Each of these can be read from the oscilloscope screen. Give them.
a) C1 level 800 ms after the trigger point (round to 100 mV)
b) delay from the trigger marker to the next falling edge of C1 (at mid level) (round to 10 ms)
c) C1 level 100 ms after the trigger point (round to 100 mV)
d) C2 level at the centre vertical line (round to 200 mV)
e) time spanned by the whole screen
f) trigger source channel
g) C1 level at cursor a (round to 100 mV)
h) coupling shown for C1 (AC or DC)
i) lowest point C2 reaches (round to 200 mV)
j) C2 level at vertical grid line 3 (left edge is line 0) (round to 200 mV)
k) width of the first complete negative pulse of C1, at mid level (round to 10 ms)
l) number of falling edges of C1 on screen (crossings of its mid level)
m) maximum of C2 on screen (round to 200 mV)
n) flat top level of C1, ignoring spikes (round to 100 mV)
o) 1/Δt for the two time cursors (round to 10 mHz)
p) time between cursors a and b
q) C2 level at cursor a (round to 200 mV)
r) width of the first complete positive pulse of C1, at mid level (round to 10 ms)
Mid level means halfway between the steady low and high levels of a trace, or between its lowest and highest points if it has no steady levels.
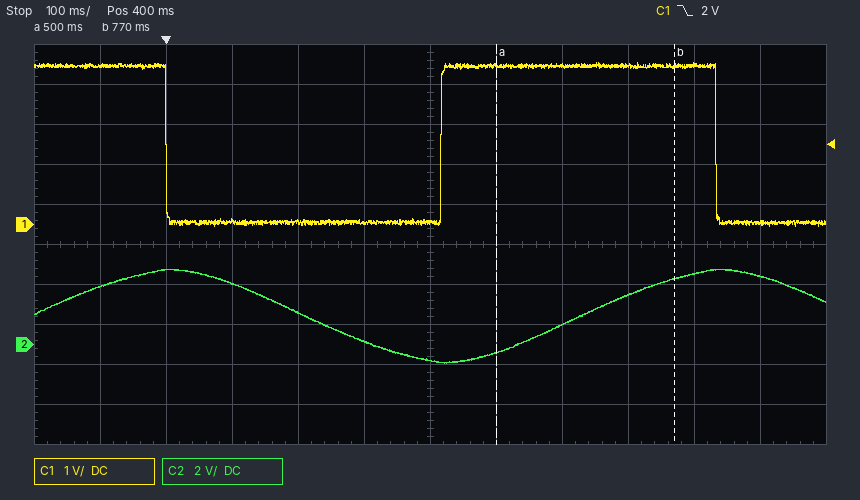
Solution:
4.0 V
830 ms
100 mV
-800 mV
1.2 s
C1
4.0 V
DC
-1.0 V
3.0 V
420 ms
2
3.8 V
4.0 V
3.70 Hz
270 ms
-400 mV
420 ms
